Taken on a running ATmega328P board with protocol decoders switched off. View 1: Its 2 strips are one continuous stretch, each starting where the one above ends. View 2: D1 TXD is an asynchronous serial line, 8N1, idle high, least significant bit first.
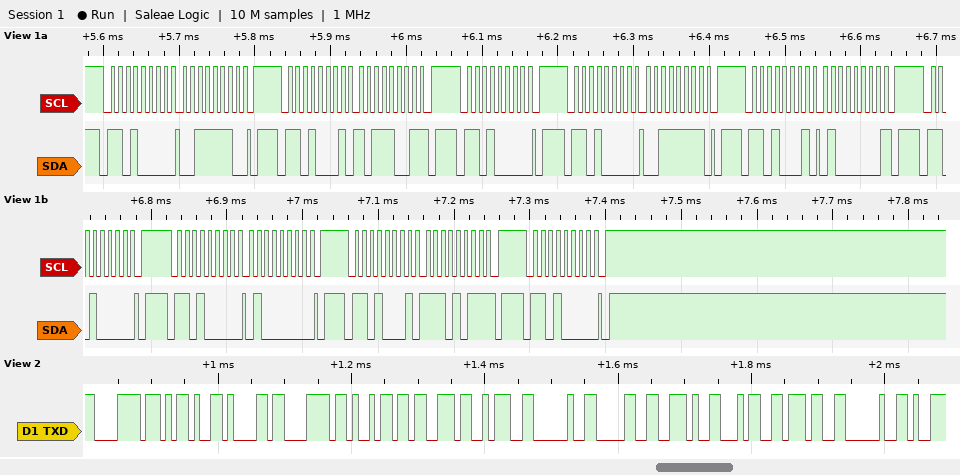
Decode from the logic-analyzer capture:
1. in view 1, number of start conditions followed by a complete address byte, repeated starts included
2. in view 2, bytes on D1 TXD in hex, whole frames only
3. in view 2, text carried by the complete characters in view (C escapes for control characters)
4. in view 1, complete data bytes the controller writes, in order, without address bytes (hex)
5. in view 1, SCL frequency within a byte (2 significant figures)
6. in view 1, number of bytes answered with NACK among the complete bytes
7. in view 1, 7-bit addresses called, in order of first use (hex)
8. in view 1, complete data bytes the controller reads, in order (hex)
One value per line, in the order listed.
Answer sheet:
9
78 2D 61 78 69 73 3A 20 30 2E 34 37 20
"x-axis: 0.47 "
3E 3F 40
100 kHz
3
0x68
B9 40 EB
